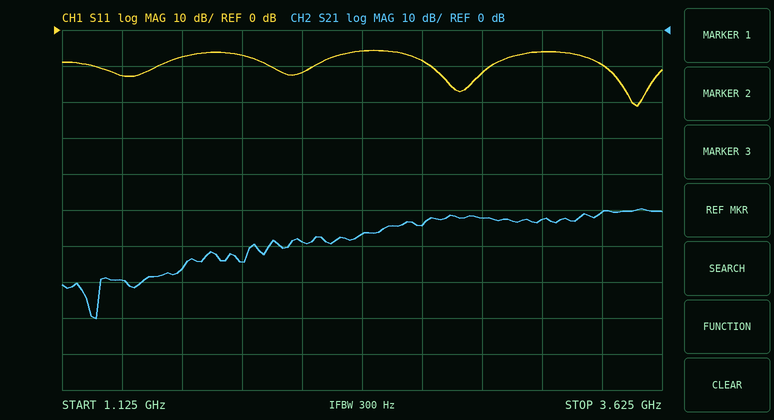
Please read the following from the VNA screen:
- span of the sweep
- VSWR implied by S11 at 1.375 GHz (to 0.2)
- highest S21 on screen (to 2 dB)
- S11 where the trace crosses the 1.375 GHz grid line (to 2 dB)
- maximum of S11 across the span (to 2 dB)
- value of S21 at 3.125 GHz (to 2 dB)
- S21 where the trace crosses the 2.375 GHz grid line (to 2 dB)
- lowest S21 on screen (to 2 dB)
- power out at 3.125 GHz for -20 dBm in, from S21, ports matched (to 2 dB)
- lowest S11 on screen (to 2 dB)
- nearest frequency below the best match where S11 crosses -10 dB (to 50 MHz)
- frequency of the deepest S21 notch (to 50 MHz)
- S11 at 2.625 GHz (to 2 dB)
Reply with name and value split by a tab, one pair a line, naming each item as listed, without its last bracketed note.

span of the sweep	2.5 GHz
VSWR implied by S11 at 1.375 GHz	1.6
highest S21 on screen	-50 dB
S11 where the trace crosses the 1.375 GHz grid line	-12 dB
maximum of S11 across the span	-6 dB
value of S21 at 3.125 GHz	-52 dB
S21 where the trace crosses the 2.375 GHz grid line	-56 dB
lowest S21 on screen	-80 dB
power out at 3.125 GHz for -20 dBm in, from S21, ports matched	-72 dBm
lowest S11 on screen	-22 dB
nearest frequency below the best match where S11 crosses -10 dB	3.40 GHz
frequency of the deepest S21 notch	1.25 GHz
S11 at 2.625 GHz	-8 dB
